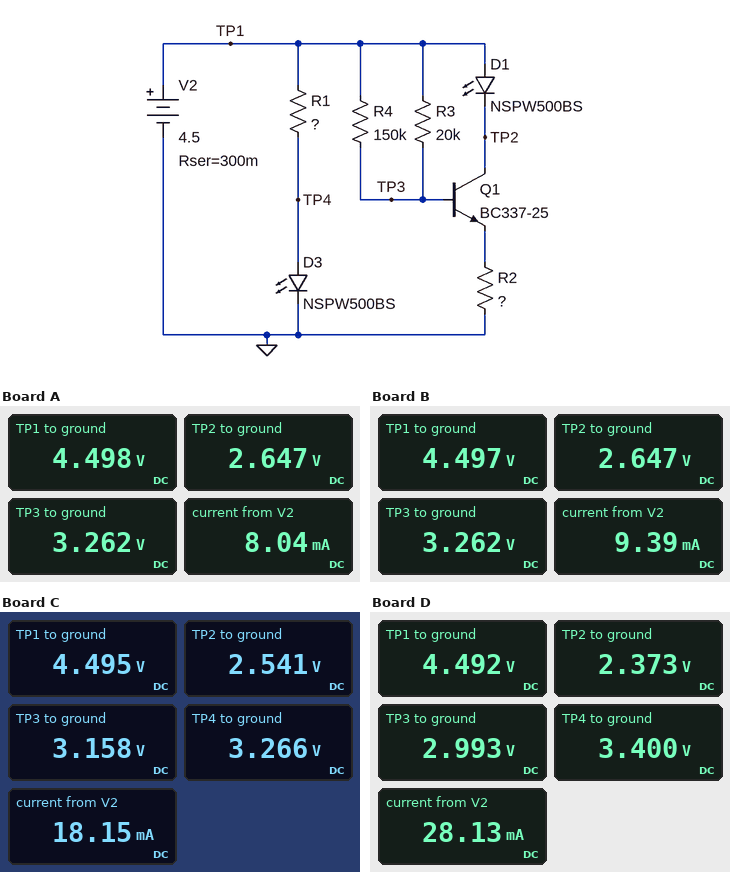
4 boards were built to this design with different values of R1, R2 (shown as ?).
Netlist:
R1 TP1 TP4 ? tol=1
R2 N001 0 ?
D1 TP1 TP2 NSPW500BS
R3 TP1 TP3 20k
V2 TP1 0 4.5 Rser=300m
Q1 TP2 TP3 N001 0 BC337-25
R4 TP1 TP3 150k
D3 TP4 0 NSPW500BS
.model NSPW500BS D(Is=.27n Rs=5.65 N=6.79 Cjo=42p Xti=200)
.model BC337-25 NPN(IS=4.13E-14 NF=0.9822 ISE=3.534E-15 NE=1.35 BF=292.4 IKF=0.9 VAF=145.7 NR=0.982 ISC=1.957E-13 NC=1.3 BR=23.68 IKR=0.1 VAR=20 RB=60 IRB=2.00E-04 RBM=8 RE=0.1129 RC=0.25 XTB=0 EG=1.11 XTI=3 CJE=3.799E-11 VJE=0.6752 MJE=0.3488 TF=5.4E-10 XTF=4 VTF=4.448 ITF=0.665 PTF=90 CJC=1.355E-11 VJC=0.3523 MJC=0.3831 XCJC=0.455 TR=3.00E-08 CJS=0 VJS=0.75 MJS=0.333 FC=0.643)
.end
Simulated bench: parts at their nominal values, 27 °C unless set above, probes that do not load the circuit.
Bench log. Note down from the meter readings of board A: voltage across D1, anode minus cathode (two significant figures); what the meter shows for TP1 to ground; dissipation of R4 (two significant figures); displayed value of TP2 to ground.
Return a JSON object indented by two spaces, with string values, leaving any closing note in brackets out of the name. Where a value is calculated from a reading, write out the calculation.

{
  "voltage across D1, anode minus cathode": "4.498 V - 2.647 V = 1.9 V",
  "what the meter shows for TP1 to ground": "4.498 V",
  "dissipation of R4": "(4.498 V - 3.262 V)^2 / 150 kΩ = 10 µW",
  "displayed value of TP2 to ground": "2.647 V"
}
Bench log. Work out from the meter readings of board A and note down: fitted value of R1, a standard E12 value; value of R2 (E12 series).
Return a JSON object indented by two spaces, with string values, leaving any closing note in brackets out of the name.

{
  "fitted value of R1, a standard E12 value": "180 Ω",
  "value of R2": "33 kΩ"
}
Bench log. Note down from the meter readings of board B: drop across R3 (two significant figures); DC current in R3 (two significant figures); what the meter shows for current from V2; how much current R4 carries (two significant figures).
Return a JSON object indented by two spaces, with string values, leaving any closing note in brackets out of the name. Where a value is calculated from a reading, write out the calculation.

{
  "drop across R3": "4.497 V - 3.262 V = 1.2 V",
  "DC current in R3": "(4.497 V - 3.262 V) / 20 kΩ = 62 µA",
  "what the meter shows for current from V2": "9.39 mA",
  "how much current R4 carries": "(4.497 V - 3.262 V) / 150 kΩ = 8.2 µA"
}
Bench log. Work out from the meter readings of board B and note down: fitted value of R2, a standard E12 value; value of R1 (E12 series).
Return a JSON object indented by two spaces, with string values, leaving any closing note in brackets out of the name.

{
  "fitted value of R2, a standard E12 value": "33 kΩ",
  "value of R1": "150 Ω"
}
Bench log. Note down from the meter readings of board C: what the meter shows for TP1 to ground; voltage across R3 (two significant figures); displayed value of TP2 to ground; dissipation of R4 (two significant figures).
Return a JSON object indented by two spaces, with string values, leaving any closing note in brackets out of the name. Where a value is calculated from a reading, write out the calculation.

{
  "what the meter shows for TP1 to ground": "4.495 V",
  "voltage across R3": "4.495 V - 3.158 V = 1.3 V",
  "displayed value of TP2 to ground": "2.541 V",
  "dissipation of R4": "(4.495 V - 3.158 V)^2 / 150 kΩ = 12 µW"
}
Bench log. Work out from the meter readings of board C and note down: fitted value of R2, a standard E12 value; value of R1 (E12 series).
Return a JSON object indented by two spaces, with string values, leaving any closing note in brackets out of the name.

{
  "fitted value of R2, a standard E12 value": "27 kΩ",
  "value of R1": "68 Ω"
}
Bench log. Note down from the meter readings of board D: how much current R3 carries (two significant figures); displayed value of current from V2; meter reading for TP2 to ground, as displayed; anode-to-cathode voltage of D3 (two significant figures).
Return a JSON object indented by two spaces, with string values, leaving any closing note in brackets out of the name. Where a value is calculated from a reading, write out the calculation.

{
  "how much current R3 carries": "(4.492 V - 2.993 V) / 20 kΩ = 75 µA",
  "displayed value of current from V2": "28.13 mA",
  "meter reading for TP2 to ground, as displayed": "2.373 V",
  "anode-to-cathode voltage of D3": "3.4 V = 3.4 V"
}
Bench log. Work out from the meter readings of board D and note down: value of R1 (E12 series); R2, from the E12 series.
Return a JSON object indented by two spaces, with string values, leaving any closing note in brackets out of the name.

{
  "value of R1": "39 Ω",
  "R2, from the E12 series": "18 kΩ"
}
